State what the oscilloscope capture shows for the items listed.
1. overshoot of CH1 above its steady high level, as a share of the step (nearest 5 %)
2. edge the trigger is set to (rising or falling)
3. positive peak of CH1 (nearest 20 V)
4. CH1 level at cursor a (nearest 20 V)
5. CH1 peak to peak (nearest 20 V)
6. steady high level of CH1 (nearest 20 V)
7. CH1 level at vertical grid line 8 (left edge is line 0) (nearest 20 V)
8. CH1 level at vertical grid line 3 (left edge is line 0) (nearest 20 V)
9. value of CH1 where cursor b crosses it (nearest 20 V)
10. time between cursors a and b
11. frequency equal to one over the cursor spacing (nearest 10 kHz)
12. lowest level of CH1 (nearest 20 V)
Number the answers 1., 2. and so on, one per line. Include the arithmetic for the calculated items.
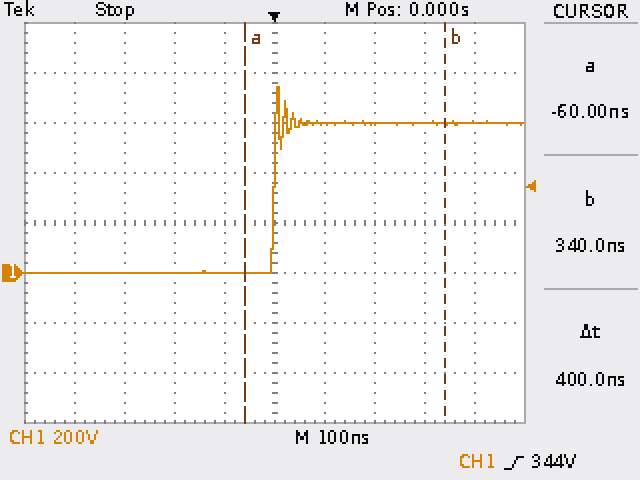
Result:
1. 25 %
2. rising
3. 740 V
4. 0 V
5. 740 V − (0 V) = 740 V
6. 600 V
7. 600 V
8. 0 V
9. 600 V
10. 400 ns
11. 1 / 400 ns ≈ 2.50 MHz
12. 0 V
